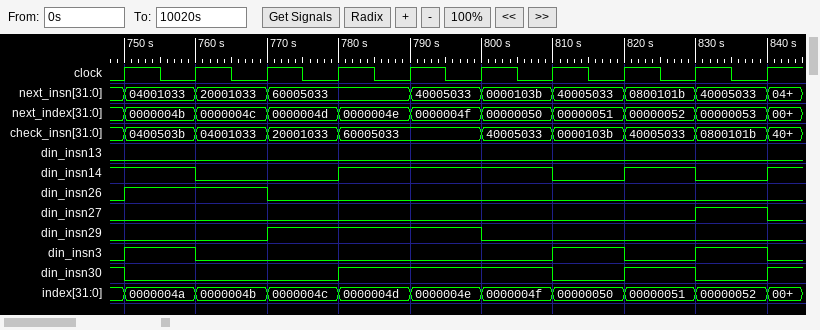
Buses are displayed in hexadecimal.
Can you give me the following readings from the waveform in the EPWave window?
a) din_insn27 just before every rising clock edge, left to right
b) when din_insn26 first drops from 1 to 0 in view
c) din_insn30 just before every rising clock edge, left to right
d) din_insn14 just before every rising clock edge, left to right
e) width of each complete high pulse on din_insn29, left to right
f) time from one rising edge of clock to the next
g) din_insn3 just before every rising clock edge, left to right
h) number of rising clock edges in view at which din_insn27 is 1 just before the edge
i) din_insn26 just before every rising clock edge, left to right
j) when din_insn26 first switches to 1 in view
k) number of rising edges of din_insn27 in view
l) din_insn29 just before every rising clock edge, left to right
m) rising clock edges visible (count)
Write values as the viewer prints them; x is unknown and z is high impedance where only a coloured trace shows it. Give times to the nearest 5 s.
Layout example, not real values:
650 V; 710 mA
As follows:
0 0 0 0 0 0 0 0 0 1; 770 s; 1 0 0 0 1 1 1 0 1 0; 1 1 0 0 1 1 1 0 1 0; 30 s; 10 s; 0 1 0 0 0 0 0 1 0 1; 1; 0 1 1 0 0 0 0 0 0 0; 750 s; 1; 0 0 0 1 1 1 0 0 0 0; 10
